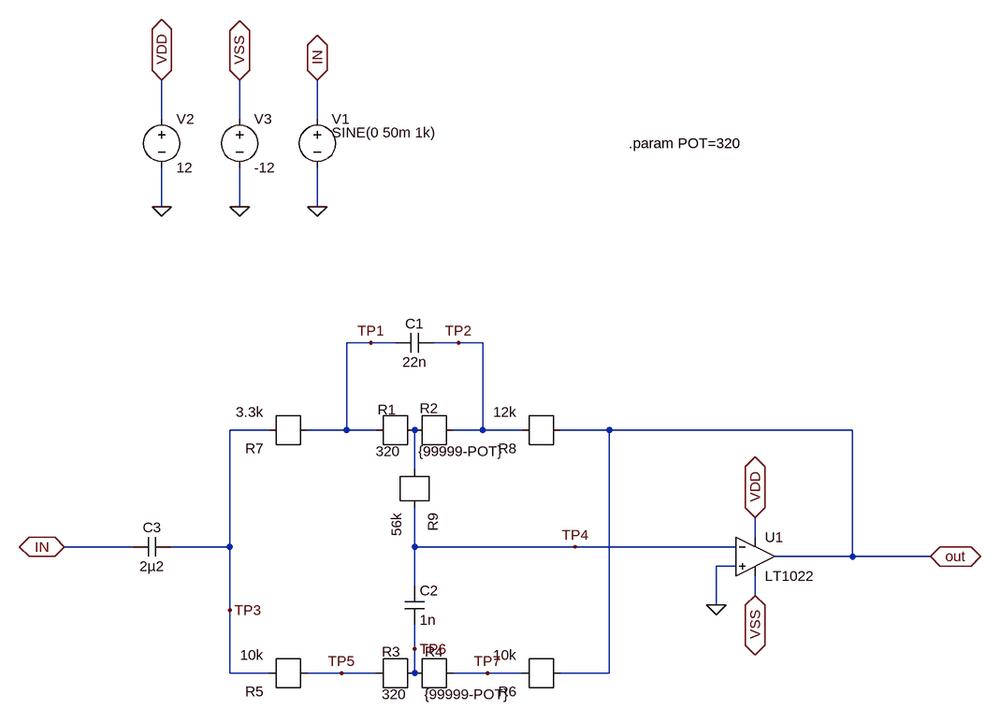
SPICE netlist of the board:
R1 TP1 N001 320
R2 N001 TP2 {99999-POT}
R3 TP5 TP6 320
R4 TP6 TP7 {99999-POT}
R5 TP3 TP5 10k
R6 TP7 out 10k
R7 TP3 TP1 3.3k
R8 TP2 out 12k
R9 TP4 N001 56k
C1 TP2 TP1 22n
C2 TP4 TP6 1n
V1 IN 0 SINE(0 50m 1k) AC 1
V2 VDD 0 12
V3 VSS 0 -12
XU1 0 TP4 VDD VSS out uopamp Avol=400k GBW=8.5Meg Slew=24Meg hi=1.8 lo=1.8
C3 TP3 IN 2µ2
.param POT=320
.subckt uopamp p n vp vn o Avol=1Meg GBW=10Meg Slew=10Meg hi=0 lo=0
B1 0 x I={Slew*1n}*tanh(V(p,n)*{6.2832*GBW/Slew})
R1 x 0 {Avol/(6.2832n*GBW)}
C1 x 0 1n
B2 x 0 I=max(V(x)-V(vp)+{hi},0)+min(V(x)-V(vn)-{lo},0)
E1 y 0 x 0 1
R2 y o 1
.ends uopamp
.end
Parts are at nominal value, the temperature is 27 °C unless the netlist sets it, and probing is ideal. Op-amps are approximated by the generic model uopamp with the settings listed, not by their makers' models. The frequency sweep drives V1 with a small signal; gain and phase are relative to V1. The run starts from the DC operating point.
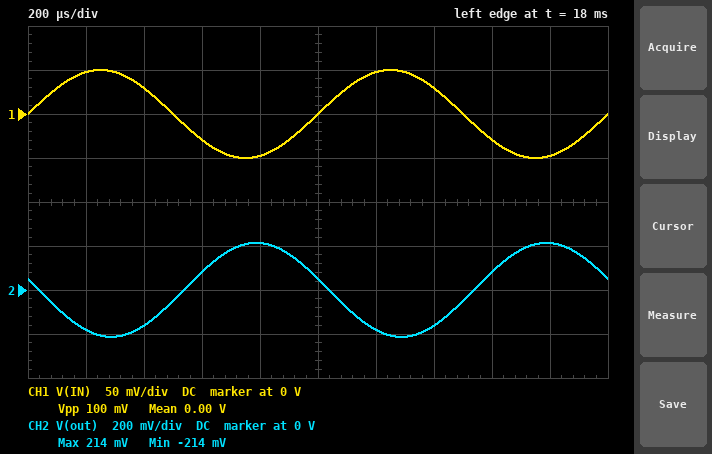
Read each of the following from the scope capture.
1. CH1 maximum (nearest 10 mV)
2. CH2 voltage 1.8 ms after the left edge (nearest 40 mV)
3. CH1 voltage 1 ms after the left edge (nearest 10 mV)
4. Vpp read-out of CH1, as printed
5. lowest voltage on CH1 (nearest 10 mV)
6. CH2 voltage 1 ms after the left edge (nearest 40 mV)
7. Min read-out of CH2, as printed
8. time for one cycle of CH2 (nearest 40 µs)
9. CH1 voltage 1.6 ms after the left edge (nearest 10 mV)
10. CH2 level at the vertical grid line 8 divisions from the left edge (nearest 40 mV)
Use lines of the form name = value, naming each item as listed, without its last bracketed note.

CH1 maximum = 50 mV
CH2 voltage 1.8 ms after the left edge = 200 mV
CH1 voltage 1 ms after the left edge = 0 V
Vpp read-out of CH1, as printed = 100 mV
lowest voltage on CH1 = -50 mV
CH2 voltage 1 ms after the left edge = 40 mV
Min read-out of CH2, as printed = -214 mV
time for one cycle of CH2 = 1.00 ms
CH1 voltage 1.6 ms after the left edge = -30 mV
CH2 level at the vertical grid line 8 divisions from the left edge = 80 mV
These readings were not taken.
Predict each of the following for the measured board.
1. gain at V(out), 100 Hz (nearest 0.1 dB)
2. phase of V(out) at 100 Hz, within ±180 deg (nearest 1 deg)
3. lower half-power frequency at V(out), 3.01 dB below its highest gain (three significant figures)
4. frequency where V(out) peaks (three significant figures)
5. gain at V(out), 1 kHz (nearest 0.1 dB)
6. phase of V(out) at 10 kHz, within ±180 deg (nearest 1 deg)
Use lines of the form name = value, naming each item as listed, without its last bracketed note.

gain at V(out), 100 Hz = 25.6 dB
phase of V(out) at 100 Hz, within ±180 deg = 154 deg
lower half-power frequency at V(out), 3.01 dB below its highest gain = 23.9 Hz
frequency where V(out) peaks = 54.0 Hz
gain at V(out), 1 kHz = 12.6 dB
phase of V(out) at 10 kHz, within ±180 deg = -167 deg
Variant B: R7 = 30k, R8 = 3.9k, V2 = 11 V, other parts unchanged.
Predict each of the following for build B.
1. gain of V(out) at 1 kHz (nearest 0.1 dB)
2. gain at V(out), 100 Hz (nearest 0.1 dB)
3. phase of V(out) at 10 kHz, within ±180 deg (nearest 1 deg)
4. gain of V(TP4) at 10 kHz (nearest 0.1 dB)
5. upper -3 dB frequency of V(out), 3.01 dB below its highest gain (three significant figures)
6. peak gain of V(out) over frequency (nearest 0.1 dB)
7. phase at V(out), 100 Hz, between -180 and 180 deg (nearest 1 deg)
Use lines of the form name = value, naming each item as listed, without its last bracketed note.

gain of V(out) at 1 kHz = -9.9 dB
gain at V(out), 100 Hz = 6.0 dB
phase of V(out) at 10 kHz, within ±180 deg = -137 deg
gain of V(TP4) at 10 kHz = -49.5 dB
upper -3 dB frequency of V(out), 3.01 dB below its highest gain = 1.67 MHz
peak gain of V(out) over frequency = 12.3 dB
phase at V(out), 100 Hz, between -180 and 180 deg = 134 deg
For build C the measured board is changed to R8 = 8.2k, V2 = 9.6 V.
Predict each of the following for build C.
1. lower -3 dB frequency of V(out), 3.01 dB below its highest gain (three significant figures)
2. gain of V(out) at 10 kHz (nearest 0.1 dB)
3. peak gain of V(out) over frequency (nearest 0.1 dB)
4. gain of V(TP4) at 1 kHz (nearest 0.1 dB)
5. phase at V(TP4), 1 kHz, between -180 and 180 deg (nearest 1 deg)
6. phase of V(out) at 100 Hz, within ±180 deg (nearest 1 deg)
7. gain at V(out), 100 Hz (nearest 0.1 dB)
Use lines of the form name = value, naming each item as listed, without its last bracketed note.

lower -3 dB frequency of V(out), 3.01 dB below its highest gain = 23.6 Hz
gain of V(out) at 10 kHz = 16.5 dB
peak gain of V(out) over frequency = 27.1 dB
gain of V(TP4) at 1 kHz = -68.2 dB
phase at V(TP4), 1 kHz, between -180 and 180 deg = 69 deg
phase of V(out) at 100 Hz, within ±180 deg = 151 deg
gain at V(out), 100 Hz = 25.3 dB
